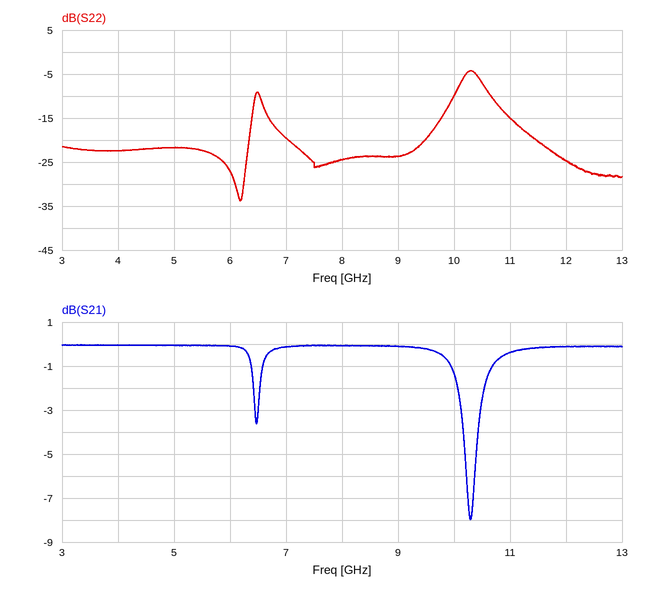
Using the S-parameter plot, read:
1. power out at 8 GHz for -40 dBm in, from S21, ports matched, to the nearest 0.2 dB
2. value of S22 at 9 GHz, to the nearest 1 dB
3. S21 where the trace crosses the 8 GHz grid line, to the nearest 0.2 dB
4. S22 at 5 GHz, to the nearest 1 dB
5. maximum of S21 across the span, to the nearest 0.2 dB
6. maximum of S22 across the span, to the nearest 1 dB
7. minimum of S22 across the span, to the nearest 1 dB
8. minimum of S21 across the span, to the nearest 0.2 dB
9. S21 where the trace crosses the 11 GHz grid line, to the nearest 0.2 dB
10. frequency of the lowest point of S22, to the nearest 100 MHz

-40.0 dBm
-24 dB
0.0 dB
-22 dB
0.0 dB
-4 dB
-34 dB
-8.0 dB
-0.4 dB
6.2 GHz
